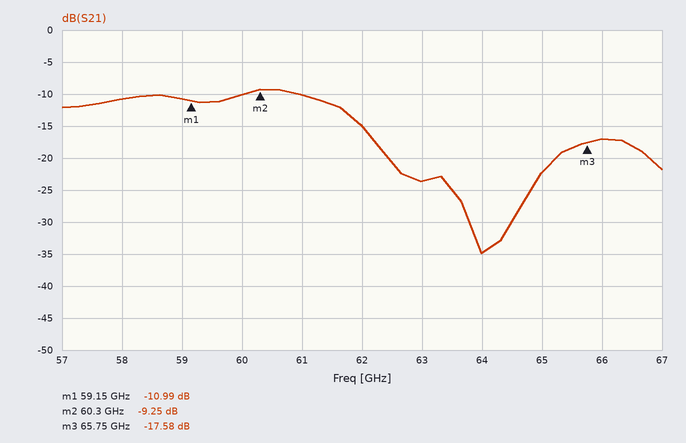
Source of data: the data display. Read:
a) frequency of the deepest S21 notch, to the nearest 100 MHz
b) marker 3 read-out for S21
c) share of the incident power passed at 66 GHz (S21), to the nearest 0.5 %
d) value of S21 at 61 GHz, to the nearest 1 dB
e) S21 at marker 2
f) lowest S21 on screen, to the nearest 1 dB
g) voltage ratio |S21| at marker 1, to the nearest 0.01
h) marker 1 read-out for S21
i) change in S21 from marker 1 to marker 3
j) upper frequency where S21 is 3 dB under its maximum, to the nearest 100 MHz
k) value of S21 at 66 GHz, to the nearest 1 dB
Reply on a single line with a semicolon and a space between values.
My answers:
64.0 GHz; -17.58 dB; 2.0 %; -10 dB; -9.25 dB; -35 dB; 0.28; -10.99 dB; -6.59 dB; 61.7 GHz; -17 dB
